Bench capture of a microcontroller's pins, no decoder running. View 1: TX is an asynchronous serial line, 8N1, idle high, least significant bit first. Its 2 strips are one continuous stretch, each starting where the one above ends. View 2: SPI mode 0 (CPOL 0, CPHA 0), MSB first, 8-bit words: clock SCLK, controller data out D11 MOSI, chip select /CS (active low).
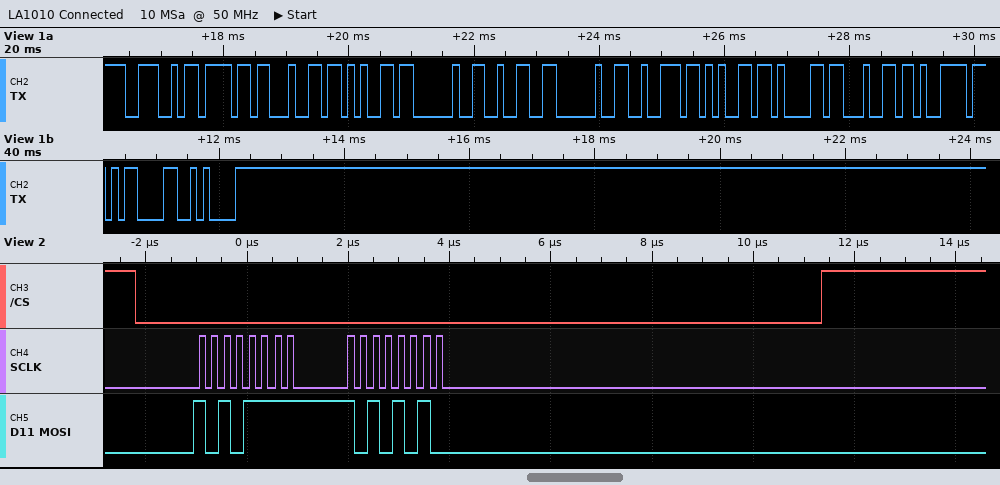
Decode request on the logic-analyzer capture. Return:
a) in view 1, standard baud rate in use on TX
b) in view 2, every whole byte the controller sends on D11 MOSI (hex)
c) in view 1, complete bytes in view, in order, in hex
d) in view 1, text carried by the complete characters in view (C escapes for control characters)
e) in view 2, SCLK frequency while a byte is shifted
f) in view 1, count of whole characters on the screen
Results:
9600 baud
AF AA
4E 6F 64 65 20 32 20 72 65 61 64 79 0D 0A
"Node 2 ready\r\n"
4 MHz
14
